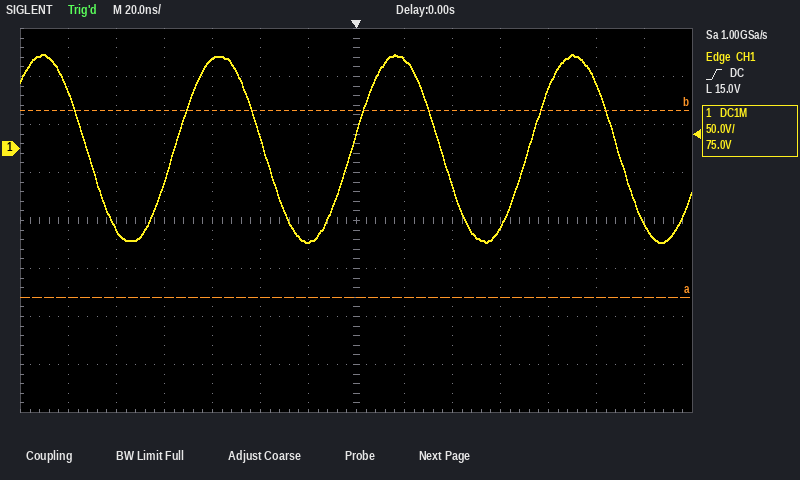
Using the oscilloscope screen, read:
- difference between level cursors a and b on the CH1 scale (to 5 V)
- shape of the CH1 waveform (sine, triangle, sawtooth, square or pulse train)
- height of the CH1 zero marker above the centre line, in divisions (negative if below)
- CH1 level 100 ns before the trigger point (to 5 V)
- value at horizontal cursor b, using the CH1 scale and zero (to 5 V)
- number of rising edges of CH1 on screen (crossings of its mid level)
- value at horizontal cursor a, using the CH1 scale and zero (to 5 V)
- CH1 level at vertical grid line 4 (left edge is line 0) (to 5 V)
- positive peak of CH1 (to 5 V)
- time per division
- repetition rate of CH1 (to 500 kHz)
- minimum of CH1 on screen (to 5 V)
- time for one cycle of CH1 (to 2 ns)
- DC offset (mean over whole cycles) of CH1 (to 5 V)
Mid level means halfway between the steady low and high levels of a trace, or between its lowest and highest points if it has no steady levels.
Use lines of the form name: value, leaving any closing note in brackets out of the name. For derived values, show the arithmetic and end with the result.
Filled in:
difference between level cursors a and b on the CH1 scale: 195 V
shape of the CH1 waveform: sine
height of the CH1 zero marker above the centre line, in divisions: +1.5 div
CH1 level 100 ns before the trigger point: -85 V
value at horizontal cursor b, using the CH1 scale and zero: 40 V
number of rising edges of CH1 on screen: 3
value at horizontal cursor a, using the CH1 scale and zero: -155 V
CH1 level at vertical grid line 4 (left edge is line 0): 95 V
positive peak of CH1: 100 V
time per division: 20 ns
repetition rate of CH1: 1 / 74 ns ≈ 13.5 MHz
minimum of CH1 on screen: -100 V
time for one cycle of CH1: 74 ns
DC offset (mean over whole cycles) of CH1: (100 V + (-100 V)) / 2 ≈ 0 V
